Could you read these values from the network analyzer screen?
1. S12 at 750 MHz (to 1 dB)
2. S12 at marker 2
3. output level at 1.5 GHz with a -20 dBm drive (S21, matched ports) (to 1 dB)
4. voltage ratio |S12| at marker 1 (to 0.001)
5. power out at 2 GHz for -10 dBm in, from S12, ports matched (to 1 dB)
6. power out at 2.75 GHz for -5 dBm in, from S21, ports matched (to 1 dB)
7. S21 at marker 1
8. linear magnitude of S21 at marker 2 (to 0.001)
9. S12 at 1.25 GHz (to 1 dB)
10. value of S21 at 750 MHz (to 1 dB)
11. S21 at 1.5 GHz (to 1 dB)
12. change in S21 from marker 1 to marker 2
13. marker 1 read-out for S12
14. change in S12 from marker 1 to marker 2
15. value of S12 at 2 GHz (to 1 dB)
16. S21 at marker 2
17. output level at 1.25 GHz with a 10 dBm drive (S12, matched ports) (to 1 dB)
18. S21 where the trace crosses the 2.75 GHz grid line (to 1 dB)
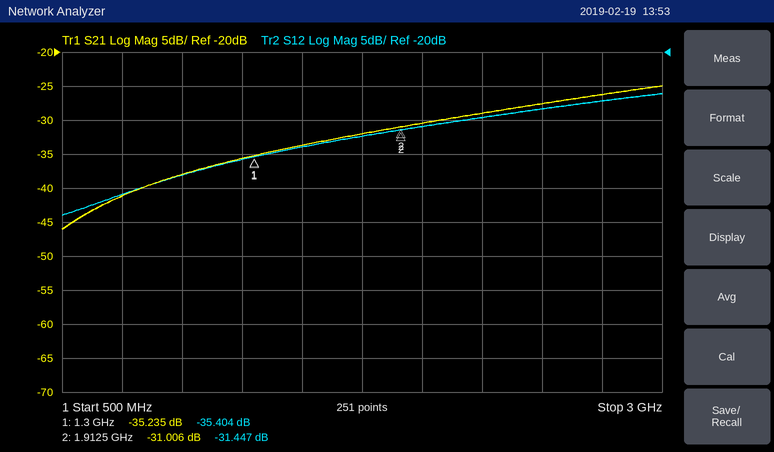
-41 dB
-31.447 dB
-54 dBm
0.017
-41 dBm
-31 dBm
-35.235 dB
0.028
-36 dB
-41 dB
-34 dB
4.229 dB
-35.404 dB
3.957 dB
-31 dB
-31.006 dB
-26 dBm
-26 dB
